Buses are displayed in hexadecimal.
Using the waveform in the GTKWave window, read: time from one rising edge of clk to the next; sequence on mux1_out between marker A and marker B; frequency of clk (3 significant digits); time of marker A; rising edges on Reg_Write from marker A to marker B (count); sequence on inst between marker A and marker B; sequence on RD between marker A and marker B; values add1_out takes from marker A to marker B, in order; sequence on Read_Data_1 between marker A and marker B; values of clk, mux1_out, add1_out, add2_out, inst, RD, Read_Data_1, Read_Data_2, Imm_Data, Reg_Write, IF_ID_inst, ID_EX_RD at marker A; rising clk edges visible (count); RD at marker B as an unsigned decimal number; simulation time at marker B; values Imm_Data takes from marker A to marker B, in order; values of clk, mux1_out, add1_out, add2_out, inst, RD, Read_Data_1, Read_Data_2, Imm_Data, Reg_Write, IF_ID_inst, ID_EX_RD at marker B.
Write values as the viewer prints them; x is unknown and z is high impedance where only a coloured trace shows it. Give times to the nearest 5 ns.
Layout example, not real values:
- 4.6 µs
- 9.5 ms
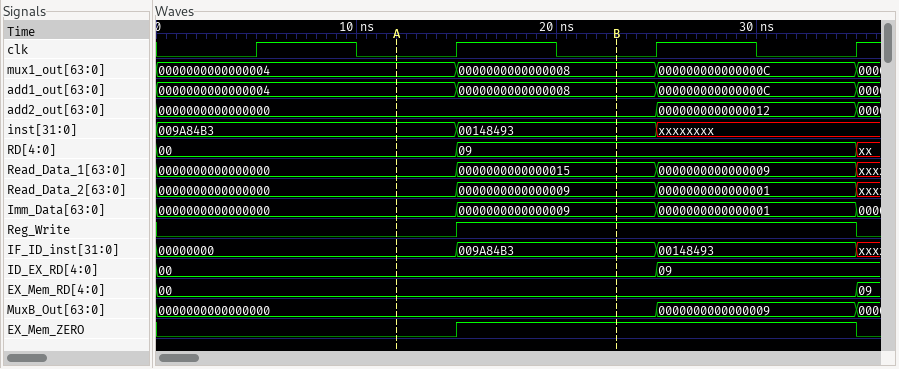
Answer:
- 10 ns
- 0000000000000004, 0000000000000008
- 100 MHz
- 10 ns
- 1
- 009A84B3, 00148493
- 00, 09
- 0000000000000004, 0000000000000008
- 0000000000000000, 0000000000000015
- clk=0, mux1_out=0000000000000004, add1_out=0000000000000004, add2_out=0000000000000000, inst=009A84B3, RD=00, Read_Data_1=0000000000000000, Read_Data_2=0000000000000000, Imm_Data=0000000000000000, Reg_Write=0, IF_ID_inst=00000000, ID_EX_RD=00
- 4
- 9
- 25 ns
- 0000000000000000, 0000000000000009
- clk=0, mux1_out=0000000000000008, add1_out=0000000000000008, add2_out=0000000000000000, inst=00148493, RD=09, Read_Data_1=0000000000000015, Read_Data_2=0000000000000009, Imm_Data=0000000000000009, Reg_Write=1, IF_ID_inst=009A84B3, ID_EX_RD=00
